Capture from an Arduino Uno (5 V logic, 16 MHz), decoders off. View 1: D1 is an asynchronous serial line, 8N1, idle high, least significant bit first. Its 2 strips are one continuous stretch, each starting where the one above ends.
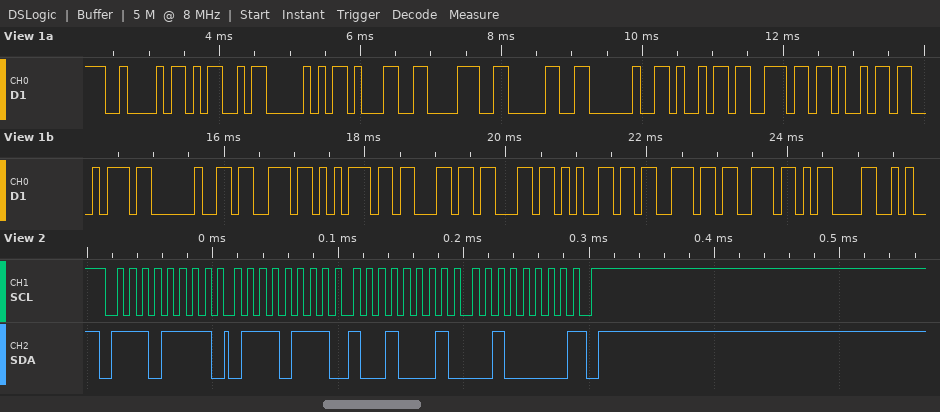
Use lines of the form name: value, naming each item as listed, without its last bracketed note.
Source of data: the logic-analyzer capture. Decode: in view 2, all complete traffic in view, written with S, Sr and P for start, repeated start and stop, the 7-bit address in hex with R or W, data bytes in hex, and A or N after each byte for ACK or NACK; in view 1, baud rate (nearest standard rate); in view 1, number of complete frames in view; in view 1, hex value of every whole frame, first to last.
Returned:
in view 2, all complete traffic in view, written with S, Sr and P for start, repeated start and stop, the 7-bit address in hex with R or W, data bytes in hex, and A or N after each byte for ACK or NACK: S 77R A 77 A 91 A 20 N P
in view 1, baud rate: 9600 baud
in view 1, number of complete frames in view: 20
in view 1, hex value of every whole frame, first to last: 42 4D 50 31 38 30 20 69 6E 69 74 20 73 75 63 63 65 73 73 0D
